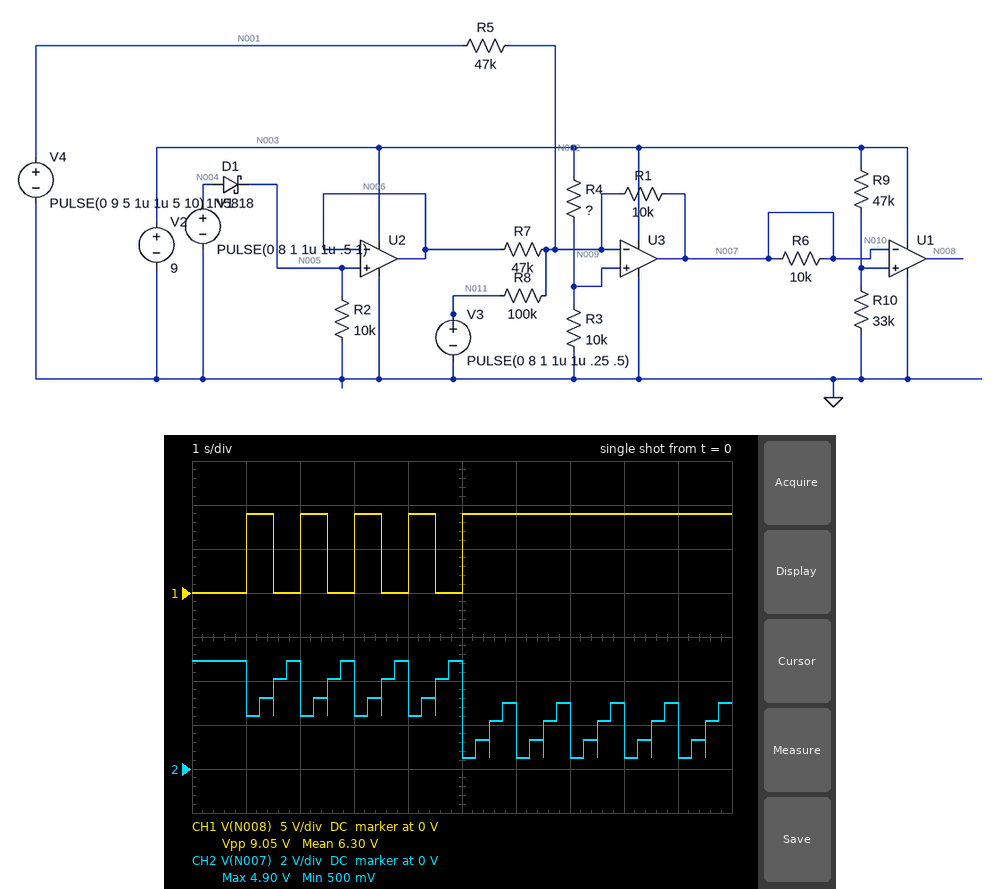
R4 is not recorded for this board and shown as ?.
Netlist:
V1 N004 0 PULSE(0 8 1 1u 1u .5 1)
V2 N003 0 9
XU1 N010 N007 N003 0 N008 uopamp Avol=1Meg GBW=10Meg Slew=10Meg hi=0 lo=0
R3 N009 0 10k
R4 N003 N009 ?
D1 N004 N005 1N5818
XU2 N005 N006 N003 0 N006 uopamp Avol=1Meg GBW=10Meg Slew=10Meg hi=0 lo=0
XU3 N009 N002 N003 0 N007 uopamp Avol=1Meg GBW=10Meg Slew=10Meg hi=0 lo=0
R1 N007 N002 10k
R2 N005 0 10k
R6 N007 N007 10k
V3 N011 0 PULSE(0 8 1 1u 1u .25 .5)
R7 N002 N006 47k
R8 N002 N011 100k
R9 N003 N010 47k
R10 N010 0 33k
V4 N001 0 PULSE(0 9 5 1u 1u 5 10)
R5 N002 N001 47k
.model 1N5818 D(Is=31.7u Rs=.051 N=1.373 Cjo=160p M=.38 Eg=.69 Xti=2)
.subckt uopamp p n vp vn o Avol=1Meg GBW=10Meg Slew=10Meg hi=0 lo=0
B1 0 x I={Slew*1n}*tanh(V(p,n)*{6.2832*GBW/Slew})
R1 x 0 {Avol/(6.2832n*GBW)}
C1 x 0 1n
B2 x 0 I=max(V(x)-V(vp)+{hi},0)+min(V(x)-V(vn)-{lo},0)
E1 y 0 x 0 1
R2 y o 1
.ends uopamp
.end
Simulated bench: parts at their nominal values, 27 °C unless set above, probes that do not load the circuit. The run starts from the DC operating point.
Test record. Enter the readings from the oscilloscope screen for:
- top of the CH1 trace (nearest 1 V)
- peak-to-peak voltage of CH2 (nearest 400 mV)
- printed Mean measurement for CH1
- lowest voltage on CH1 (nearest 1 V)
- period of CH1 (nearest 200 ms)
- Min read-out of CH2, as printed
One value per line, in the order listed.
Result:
9 V
4.4 V
6.30 V
0 V
1.0 s
500 mV
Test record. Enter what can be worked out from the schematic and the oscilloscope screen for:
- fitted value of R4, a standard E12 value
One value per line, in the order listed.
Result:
18 kΩ
